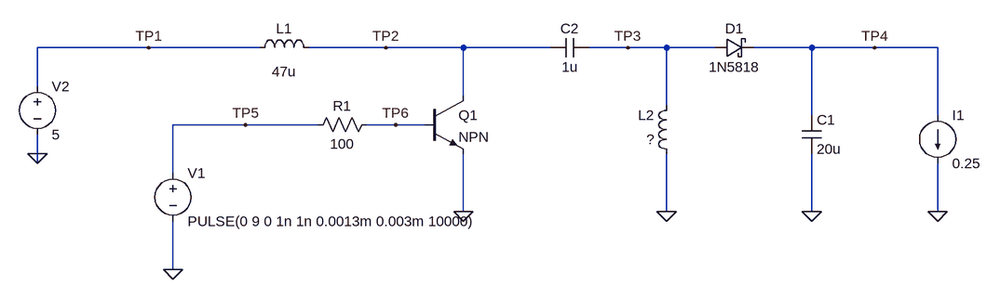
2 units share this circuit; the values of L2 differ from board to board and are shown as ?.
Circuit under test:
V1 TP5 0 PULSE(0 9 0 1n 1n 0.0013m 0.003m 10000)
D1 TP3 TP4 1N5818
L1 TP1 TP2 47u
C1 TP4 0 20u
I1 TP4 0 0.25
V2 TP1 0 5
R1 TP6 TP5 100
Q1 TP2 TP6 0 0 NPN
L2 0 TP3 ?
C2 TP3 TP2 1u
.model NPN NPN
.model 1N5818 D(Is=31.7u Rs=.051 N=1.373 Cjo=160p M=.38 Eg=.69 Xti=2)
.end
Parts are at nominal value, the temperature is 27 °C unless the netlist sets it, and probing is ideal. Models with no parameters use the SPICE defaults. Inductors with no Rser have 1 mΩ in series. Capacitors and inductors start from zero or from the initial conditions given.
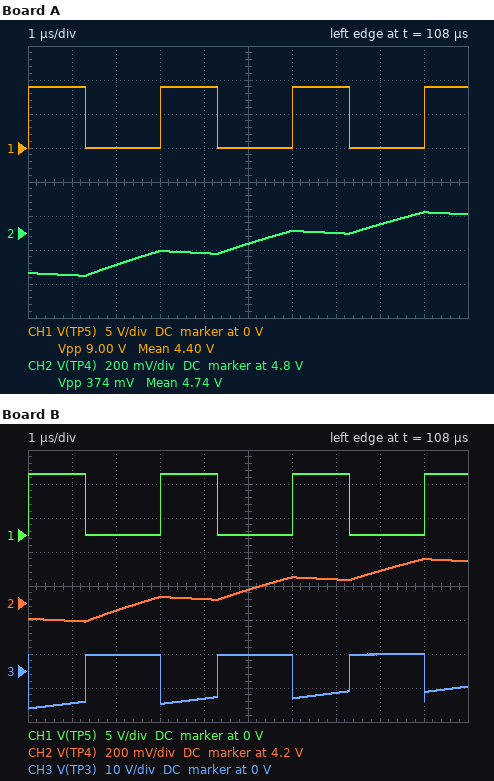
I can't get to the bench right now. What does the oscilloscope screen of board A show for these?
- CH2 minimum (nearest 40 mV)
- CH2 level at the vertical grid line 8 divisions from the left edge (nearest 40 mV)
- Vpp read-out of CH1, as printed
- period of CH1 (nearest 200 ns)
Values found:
4.56 V
4.84 V
9.00 V
3.0 µs
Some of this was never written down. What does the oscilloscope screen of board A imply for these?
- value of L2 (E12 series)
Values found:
100 µH
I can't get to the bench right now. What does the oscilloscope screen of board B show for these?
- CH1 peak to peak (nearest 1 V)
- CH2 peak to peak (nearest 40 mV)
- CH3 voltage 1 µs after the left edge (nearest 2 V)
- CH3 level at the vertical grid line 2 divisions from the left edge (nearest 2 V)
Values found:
9 V
360 mV
-10 V
4 V
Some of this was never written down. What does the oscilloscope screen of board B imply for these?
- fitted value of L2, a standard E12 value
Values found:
120 µH
